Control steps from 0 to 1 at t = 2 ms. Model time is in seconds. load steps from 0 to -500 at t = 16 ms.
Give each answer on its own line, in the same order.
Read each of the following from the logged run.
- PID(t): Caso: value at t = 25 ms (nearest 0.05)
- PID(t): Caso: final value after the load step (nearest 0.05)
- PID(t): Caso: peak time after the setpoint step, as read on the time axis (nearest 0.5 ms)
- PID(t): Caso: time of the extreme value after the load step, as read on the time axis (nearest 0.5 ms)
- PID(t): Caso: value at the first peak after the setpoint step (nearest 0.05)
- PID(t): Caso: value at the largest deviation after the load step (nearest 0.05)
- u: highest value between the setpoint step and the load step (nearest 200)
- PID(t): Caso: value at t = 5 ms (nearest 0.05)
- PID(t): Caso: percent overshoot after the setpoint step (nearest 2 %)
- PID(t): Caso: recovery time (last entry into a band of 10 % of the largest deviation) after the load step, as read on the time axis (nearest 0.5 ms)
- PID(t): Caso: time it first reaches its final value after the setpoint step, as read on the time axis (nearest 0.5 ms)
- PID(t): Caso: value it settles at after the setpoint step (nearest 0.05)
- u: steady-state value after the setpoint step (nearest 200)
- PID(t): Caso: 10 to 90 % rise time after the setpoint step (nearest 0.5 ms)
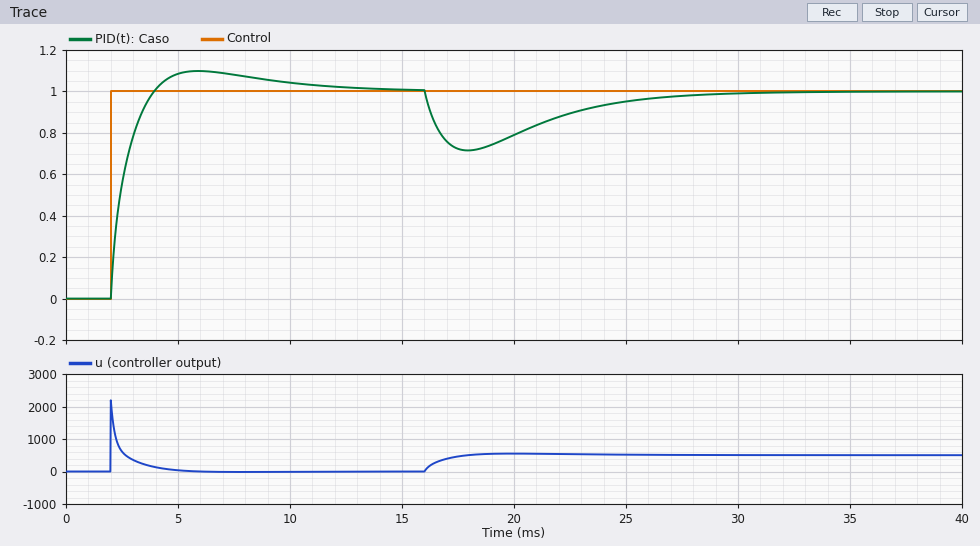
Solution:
0.95
1.00
6.0 ms
18.0 ms
1.10
0.70
2200
1.10
10 %
26.5 ms
4.0 ms
1.00
0
1.5 ms
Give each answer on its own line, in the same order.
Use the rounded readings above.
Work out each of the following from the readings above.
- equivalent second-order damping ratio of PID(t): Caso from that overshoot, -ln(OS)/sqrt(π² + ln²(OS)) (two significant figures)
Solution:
0.59
